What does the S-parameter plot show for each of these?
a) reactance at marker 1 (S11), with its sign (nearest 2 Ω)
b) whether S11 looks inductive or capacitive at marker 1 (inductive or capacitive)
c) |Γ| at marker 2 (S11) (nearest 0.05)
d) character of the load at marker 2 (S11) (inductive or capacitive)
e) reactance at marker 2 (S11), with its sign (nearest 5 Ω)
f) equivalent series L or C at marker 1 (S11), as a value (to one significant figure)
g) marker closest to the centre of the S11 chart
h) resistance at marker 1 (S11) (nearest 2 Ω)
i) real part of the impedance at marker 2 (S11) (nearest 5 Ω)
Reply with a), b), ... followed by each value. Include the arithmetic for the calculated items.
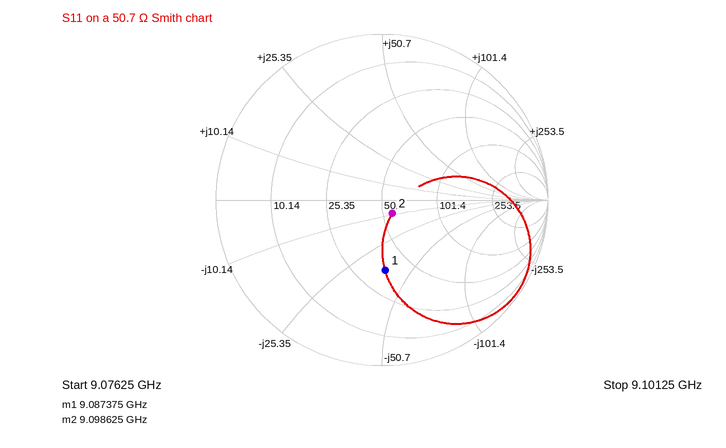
a) -38 Ω
b) capacitive
c) 0.10
d) capacitive
e) -10 Ω
f) C = 1/(2π × 9.087375 GHz × 38 Ω) ≈ 461 fF, so 500 fF to one significant figure
g) marker 2
h) 36 Ω
i) 55 Ω
